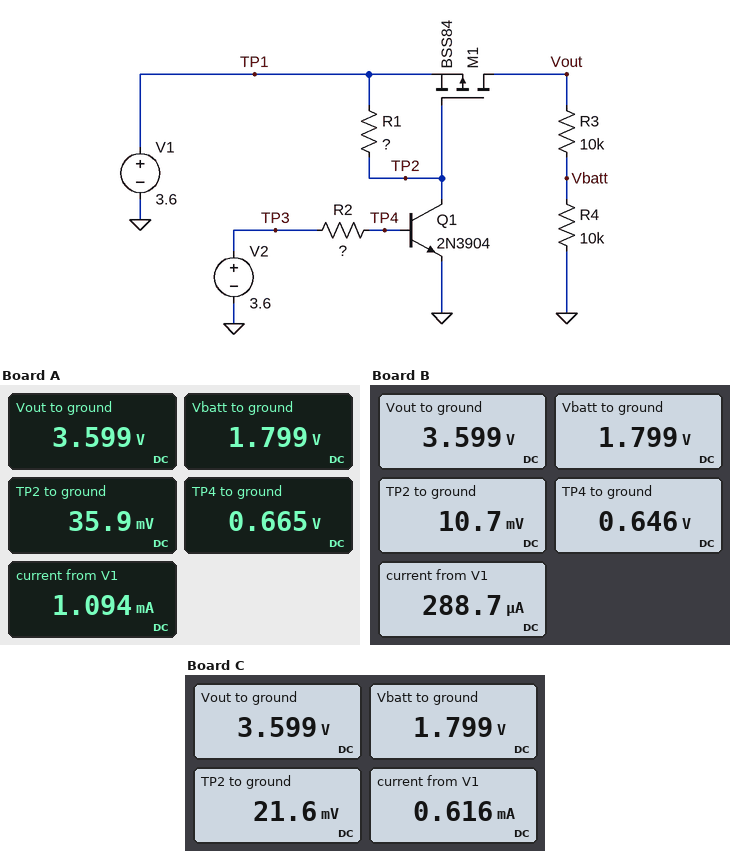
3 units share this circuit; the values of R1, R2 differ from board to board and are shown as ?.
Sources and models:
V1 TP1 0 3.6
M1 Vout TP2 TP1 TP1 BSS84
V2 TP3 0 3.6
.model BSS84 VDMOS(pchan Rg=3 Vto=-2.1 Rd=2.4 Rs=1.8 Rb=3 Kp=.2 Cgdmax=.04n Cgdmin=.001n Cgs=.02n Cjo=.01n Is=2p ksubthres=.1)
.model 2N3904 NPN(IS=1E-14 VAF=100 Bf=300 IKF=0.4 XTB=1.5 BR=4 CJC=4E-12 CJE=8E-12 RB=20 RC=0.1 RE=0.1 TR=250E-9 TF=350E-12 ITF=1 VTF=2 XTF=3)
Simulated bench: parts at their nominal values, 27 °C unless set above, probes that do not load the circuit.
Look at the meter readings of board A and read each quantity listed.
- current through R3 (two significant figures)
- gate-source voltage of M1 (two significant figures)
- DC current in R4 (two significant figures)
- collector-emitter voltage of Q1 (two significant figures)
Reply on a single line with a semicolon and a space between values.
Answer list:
180 µA; -3.6 V; 180 µA; 36 mV
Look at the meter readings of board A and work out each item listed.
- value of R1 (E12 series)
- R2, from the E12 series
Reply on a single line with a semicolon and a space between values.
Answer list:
3.9 kΩ; 33 kΩ
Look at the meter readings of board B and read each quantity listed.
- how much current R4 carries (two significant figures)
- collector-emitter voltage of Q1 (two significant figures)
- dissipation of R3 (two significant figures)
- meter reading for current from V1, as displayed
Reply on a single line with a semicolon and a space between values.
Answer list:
180 µA; 11 mV; 320 µW; 288.7 µA
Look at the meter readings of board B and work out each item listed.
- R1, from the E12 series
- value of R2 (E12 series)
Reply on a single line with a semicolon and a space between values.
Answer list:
33 kΩ; 27 kΩ
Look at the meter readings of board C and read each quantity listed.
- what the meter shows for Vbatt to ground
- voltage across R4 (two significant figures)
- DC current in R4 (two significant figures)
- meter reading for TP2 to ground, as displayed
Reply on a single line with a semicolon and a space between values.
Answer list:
1.799 V; 1.8 V; 180 µA; 21.6 mV
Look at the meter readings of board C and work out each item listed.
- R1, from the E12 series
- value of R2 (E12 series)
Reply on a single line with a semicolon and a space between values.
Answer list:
8.2 kΩ; 27 kΩ
